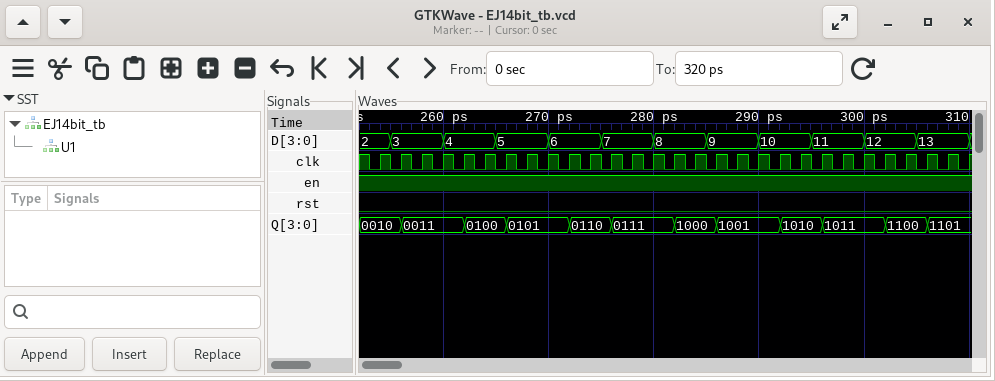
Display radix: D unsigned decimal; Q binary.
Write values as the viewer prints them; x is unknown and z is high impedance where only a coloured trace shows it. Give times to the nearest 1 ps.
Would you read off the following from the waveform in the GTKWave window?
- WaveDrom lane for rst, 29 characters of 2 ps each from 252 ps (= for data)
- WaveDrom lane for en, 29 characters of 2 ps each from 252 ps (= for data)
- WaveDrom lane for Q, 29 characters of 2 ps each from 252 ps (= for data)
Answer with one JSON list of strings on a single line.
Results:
["{name: 'rst', wave: '0............................'}", "{name: 'en', wave: '1............................'}", "{name: 'Q', wave: '=.=..=.=..=.=..=.=..=.=..=.=.', data: '0010 0011 0100 0101 0110 0111 1000 1001 1010 1011 1100 1101'}"]
